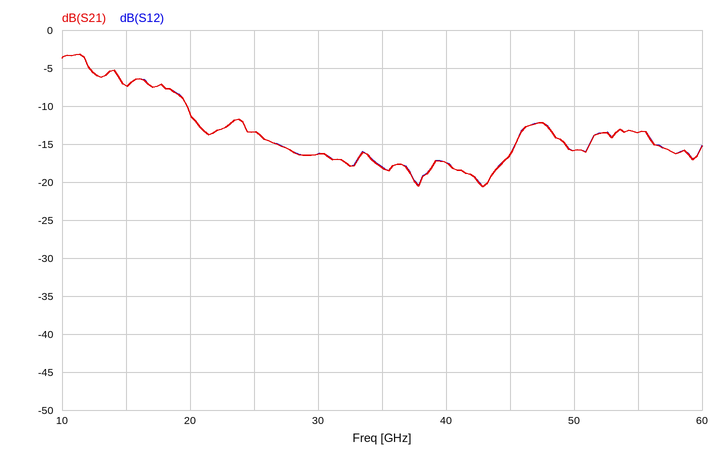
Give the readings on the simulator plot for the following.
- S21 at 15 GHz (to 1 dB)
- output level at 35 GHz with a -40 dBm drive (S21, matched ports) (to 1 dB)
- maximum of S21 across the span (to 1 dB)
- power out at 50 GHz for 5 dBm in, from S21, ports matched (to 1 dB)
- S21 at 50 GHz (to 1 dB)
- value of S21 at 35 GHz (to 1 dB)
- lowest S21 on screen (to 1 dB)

-7 dB
-58 dBm
-3 dB
-11 dBm
-16 dB
-18 dB
-21 dB
